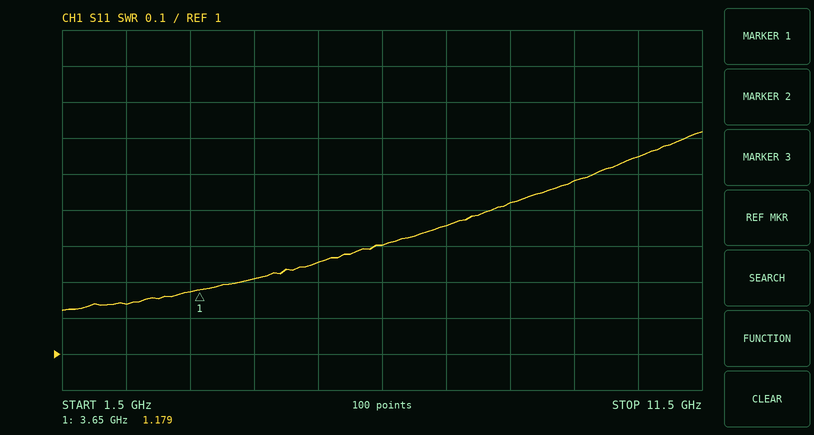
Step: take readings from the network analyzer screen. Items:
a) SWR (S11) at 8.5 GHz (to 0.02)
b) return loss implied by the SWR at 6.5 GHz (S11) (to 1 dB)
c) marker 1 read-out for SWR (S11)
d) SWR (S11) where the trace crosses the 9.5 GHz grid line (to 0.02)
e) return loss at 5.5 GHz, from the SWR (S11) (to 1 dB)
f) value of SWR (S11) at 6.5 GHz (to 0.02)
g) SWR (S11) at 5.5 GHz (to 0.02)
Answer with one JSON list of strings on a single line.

["1.42", "18 dB", "1.179", "1.48", "19 dB", "1.30", "1.26"]
